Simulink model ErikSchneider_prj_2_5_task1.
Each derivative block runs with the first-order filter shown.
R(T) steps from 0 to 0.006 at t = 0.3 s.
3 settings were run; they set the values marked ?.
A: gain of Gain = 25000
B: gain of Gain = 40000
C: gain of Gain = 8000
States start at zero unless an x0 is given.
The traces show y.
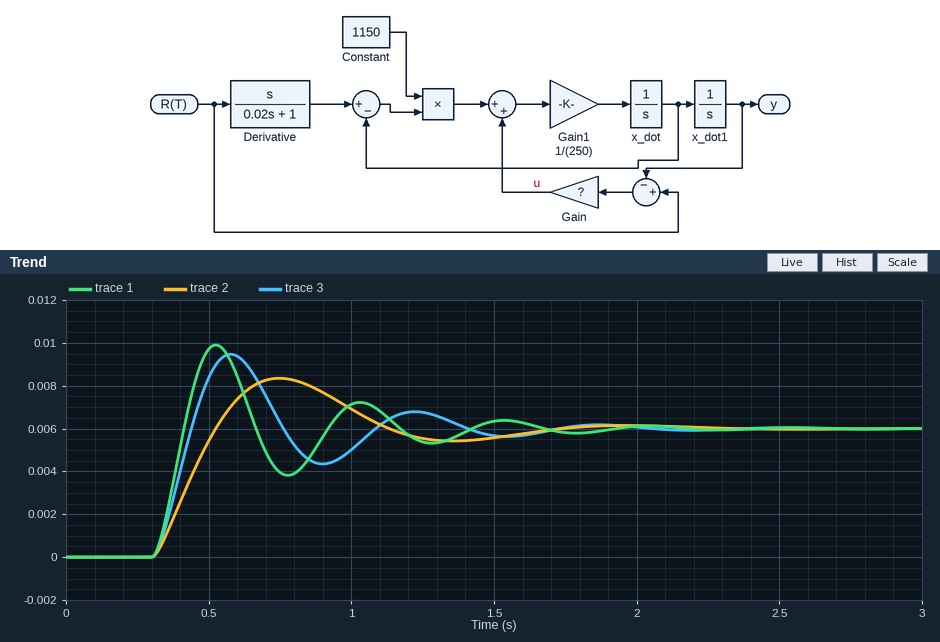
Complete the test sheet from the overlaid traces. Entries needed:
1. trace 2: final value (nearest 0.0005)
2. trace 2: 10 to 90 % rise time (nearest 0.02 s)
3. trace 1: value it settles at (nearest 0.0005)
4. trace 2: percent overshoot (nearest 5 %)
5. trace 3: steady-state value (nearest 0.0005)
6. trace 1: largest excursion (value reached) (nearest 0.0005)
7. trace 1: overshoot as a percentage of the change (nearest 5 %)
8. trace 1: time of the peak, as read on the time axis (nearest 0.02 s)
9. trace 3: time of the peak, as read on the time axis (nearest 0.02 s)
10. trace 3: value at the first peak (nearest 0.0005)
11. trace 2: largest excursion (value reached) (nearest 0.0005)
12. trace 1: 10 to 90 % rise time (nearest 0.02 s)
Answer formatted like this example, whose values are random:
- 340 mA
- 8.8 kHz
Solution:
- 0.0060
- 0.16 s
- 0.0060
- 40 %
- 0.0060
- 0.0100
- 65 %
- 0.52 s
- 0.58 s
- 0.0095
- 0.0085
- 0.08 s
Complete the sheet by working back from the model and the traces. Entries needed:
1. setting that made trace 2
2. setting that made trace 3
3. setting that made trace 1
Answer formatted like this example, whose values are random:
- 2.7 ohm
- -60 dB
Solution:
- C
- A
- B
